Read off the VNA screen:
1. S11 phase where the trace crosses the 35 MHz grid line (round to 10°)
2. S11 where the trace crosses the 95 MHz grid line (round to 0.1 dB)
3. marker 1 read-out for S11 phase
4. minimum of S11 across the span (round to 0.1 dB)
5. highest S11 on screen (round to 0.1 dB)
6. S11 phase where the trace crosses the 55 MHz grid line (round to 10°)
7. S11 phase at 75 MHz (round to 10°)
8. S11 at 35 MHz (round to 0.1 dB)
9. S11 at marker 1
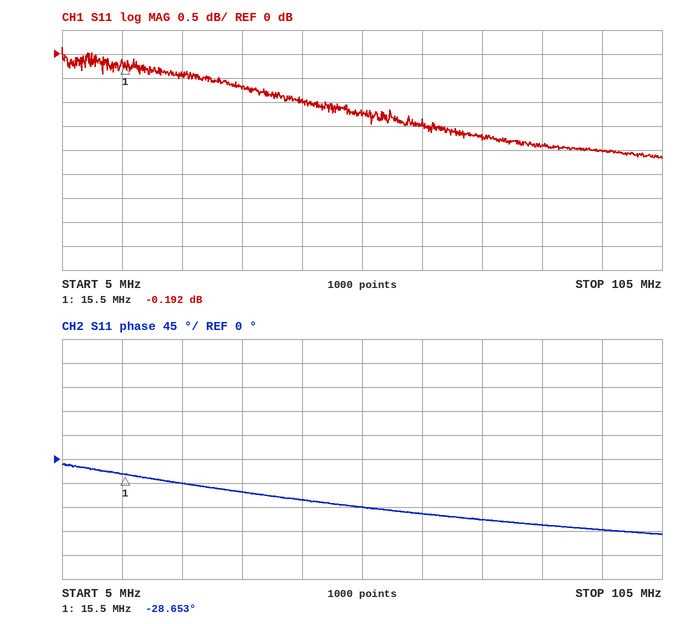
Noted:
-60°
-2.0 dB
-28.653°
-2.2 dB
0.1 dB
-90°
-110°
-0.7 dB
-0.192 dB
